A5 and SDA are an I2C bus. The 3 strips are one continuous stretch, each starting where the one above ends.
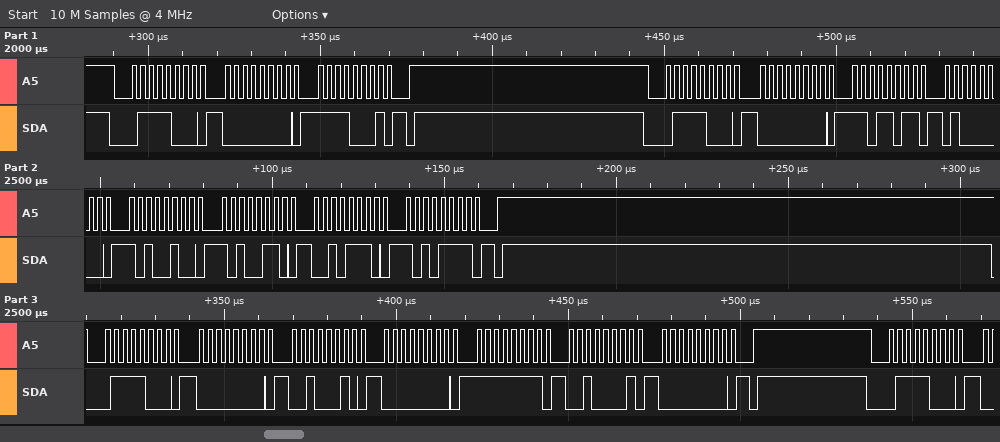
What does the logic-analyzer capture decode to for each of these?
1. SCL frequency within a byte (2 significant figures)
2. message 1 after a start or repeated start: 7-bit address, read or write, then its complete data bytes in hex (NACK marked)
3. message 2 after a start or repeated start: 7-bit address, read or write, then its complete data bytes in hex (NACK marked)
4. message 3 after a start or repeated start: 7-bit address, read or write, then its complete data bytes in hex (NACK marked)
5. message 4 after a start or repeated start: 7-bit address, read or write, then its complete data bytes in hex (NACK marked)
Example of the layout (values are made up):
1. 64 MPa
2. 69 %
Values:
1. 400 kHz
2. 0x3C write: 00 F1
3. 0x3C write: 00 DB 40 A4 A6 2E AF
4. 0x3C write: 00 22 00 FF 21 00
5. 0x3C write
